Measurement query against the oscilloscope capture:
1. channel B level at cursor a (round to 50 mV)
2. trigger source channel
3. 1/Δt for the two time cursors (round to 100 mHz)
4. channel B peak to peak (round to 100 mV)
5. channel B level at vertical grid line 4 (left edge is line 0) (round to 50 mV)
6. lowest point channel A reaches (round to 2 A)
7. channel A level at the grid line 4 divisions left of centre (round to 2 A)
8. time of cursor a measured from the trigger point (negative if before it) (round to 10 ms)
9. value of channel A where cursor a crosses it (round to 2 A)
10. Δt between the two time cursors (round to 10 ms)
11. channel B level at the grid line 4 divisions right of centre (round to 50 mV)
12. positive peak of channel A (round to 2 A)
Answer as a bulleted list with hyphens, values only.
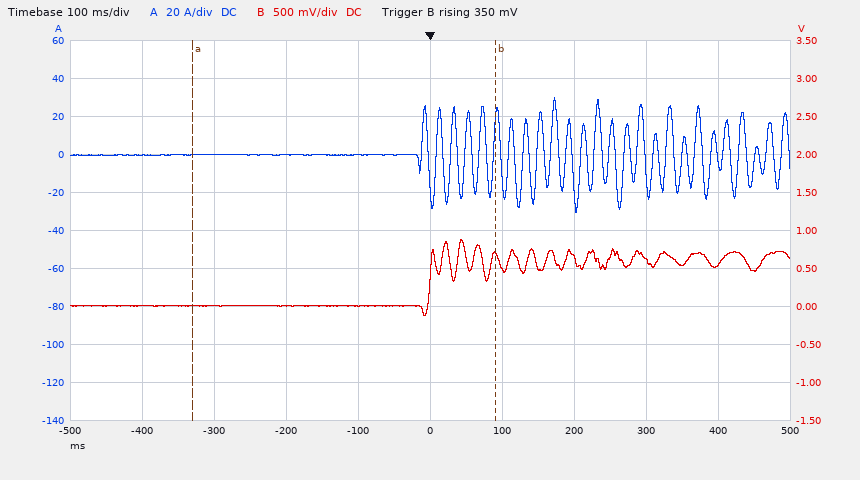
- 0 mV
- channel B
- 2.4 Hz
- 1.00 V
- 0 mV
- -30 A
- 0 A
- -330 ms
- 0 A
- 420 ms
- 550 mV
- 30 A
